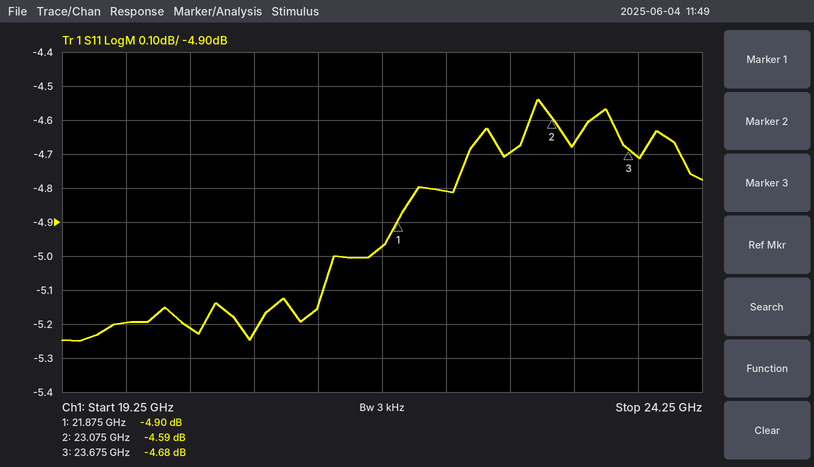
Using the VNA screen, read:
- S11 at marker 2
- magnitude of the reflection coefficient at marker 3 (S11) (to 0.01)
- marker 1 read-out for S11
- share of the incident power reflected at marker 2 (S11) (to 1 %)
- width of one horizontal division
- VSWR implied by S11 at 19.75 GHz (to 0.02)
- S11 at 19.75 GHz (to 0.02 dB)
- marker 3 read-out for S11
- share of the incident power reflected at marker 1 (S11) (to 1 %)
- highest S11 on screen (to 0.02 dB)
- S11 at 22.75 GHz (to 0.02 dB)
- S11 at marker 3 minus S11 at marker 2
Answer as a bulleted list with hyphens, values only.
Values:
- -4.59 dB
- 0.58
- -4.90 dB
- 35 %
- 500 MHz
- 3.44
- -5.20 dB
- -4.68 dB
- 32 %
- -4.54 dB
- -4.70 dB
- -0.09 dB
